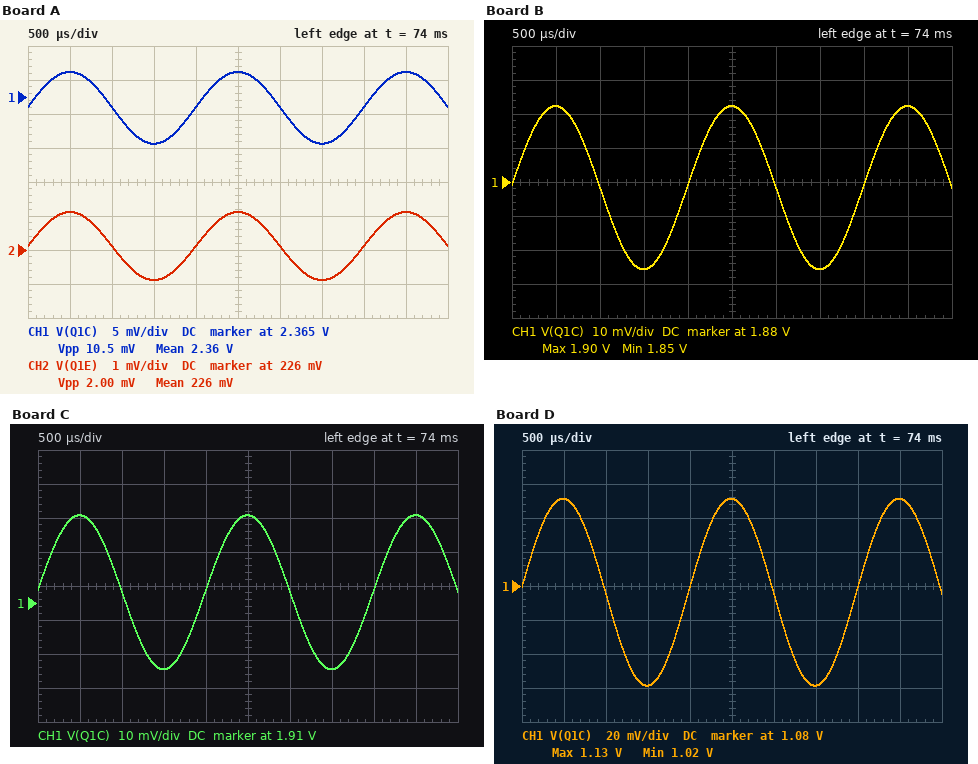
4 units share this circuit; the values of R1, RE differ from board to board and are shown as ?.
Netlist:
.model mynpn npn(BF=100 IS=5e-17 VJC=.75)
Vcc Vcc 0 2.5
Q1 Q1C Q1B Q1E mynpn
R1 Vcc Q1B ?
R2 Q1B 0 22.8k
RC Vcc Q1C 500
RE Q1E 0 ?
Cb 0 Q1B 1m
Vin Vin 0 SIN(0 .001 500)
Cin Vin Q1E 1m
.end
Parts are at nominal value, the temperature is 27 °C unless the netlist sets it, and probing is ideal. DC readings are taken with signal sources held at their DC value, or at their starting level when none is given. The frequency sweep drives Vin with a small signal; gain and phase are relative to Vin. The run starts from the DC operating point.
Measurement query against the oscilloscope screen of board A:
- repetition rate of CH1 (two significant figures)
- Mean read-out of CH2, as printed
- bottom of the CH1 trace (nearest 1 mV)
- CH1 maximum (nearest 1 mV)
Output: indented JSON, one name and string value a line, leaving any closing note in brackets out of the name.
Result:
{
  "repetition rate of CH1": "500 Hz",
  "Mean read-out of CH2, as printed": "226 mV",
  "bottom of the CH1 trace": "2.358 V",
  "CH1 maximum": "2.369 V"
}
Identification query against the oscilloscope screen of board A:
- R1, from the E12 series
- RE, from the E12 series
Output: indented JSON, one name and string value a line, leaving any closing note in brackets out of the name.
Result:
{
  "R1, from the E12 series": "33 kΩ",
  "RE, from the E12 series": "820 Ω"
}
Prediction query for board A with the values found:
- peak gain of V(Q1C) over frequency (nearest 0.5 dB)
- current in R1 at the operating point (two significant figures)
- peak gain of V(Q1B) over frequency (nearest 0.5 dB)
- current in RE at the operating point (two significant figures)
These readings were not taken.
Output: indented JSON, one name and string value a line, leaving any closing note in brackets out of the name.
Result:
{
  "peak gain of V(Q1C) over frequency": "14.5 dB",
  "current in R1 at the operating point": "46 µA",
  "peak gain of V(Q1B) over frequency": "-41.0 dB",
  "current in RE at the operating point": "280 µA"
}
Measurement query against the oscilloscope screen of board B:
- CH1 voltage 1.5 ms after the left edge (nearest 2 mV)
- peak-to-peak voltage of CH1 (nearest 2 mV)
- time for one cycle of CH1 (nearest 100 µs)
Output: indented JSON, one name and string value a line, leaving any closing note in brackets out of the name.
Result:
{
  "CH1 voltage 1.5 ms after the left edge": "1.854 V",
  "peak-to-peak voltage of CH1": "48 mV",
  "time for one cycle of CH1": "2.0 ms"
}
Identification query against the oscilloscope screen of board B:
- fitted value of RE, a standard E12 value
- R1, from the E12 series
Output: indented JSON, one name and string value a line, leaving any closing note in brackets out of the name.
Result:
{
  "fitted value of RE, a standard E12 value": "680 Ω",
  "R1, from the E12 series": "10 kΩ"
}
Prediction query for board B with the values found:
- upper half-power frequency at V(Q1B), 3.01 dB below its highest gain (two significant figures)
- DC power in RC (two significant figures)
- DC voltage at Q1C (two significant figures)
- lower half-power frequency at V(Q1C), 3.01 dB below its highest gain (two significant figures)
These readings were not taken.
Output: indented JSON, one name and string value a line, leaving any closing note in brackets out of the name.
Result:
{
  "upper half-power frequency at V(Q1B), 3.01 dB below its highest gain": "8.1 Hz",
  "DC power in RC": "770 µW",
  "DC voltage at Q1C": "1.9 V",
  "lower half-power frequency at V(Q1C), 3.01 dB below its highest gain": "8.0 Hz"
}
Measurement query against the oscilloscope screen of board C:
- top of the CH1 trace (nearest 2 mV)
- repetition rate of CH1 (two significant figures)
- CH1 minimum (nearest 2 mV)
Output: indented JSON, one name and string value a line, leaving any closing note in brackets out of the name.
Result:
{
  "top of the CH1 trace": "1.936 V",
  "repetition rate of CH1": "500 Hz",
  "CH1 minimum": "1.890 V"
}
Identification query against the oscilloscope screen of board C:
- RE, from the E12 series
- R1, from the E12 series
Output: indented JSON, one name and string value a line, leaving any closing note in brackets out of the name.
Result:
{
  "RE, from the E12 series": "820 Ω",
  "R1, from the E12 series": "8.2 kΩ"
}
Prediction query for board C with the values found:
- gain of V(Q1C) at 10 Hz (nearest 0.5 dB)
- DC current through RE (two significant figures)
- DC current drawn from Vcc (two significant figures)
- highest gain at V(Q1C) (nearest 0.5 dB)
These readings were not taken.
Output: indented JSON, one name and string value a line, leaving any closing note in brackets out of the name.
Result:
{
  "gain of V(Q1C) at 10 Hz": "25.0 dB",
  "DC current through RE": "1.2 mA",
  "DC current drawn from Vcc": "1.3 mA",
  "highest gain at V(Q1C)": "27.0 dB"
}
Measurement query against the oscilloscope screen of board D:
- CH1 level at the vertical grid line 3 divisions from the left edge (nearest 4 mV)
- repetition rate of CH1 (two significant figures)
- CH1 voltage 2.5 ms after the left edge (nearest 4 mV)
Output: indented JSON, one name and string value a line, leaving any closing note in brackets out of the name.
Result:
{
  "CH1 level at the vertical grid line 3 divisions from the left edge": "1.020 V",
  "repetition rate of CH1": "500 Hz",
  "CH1 voltage 2.5 ms after the left edge": "1.132 V"
}
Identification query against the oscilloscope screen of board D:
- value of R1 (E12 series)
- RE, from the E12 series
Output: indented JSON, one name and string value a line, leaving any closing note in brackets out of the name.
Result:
{
  "value of R1": "15 kΩ",
  "RE, from the E12 series": "150 Ω"
}
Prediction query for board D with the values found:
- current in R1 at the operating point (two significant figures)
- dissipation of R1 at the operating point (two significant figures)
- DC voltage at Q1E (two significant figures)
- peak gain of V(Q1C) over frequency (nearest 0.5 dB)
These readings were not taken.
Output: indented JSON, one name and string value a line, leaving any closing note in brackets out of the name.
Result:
{
  "current in R1 at the operating point": "83 µA",
  "dissipation of R1 at the operating point": "100 µW",
  "DC voltage at Q1E": "430 mV",
  "peak gain of V(Q1C) over frequency": "35.0 dB"
}
